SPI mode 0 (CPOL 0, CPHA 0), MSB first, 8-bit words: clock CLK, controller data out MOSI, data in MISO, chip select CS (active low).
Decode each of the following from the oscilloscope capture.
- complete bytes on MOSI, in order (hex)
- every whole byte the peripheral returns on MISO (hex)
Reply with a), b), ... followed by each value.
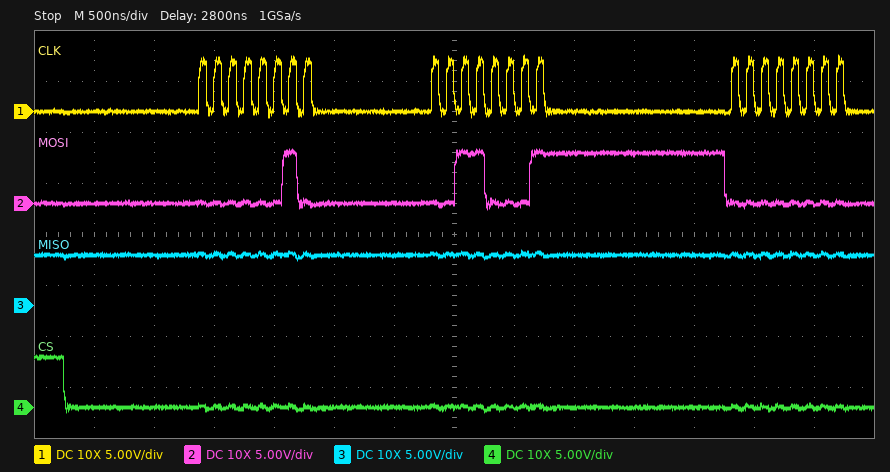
a) 0x02 0x31 0x00
b) 0xFF 0xFF 0xFF
